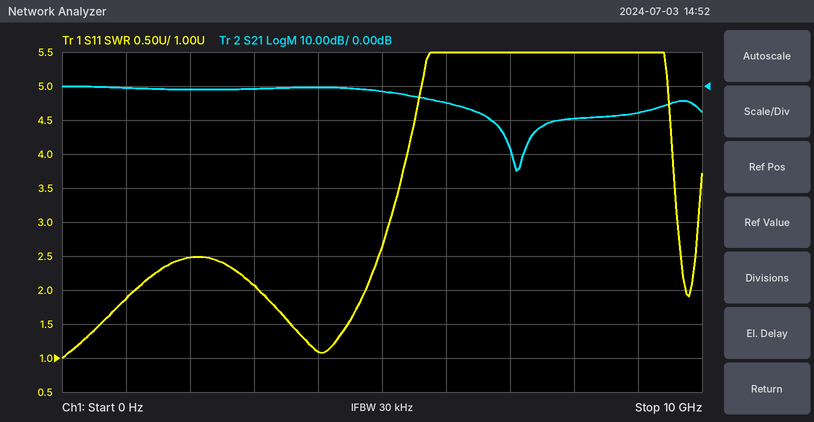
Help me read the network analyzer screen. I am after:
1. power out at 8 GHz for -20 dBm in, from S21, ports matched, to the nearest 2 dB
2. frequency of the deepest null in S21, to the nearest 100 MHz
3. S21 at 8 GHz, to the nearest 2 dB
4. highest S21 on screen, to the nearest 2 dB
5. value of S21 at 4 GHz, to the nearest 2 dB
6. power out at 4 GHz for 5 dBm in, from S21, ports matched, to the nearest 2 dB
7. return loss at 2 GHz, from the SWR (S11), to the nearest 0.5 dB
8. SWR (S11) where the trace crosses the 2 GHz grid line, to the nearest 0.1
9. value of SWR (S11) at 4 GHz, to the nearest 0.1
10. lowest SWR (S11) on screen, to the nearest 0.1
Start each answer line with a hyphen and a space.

- -30 dBm
- 7.1 GHz
- -10 dB
- 0 dB
- 0 dB
- 4 dBm
- 7.5 dB
- 2.5
- 1.1
- 1.0
